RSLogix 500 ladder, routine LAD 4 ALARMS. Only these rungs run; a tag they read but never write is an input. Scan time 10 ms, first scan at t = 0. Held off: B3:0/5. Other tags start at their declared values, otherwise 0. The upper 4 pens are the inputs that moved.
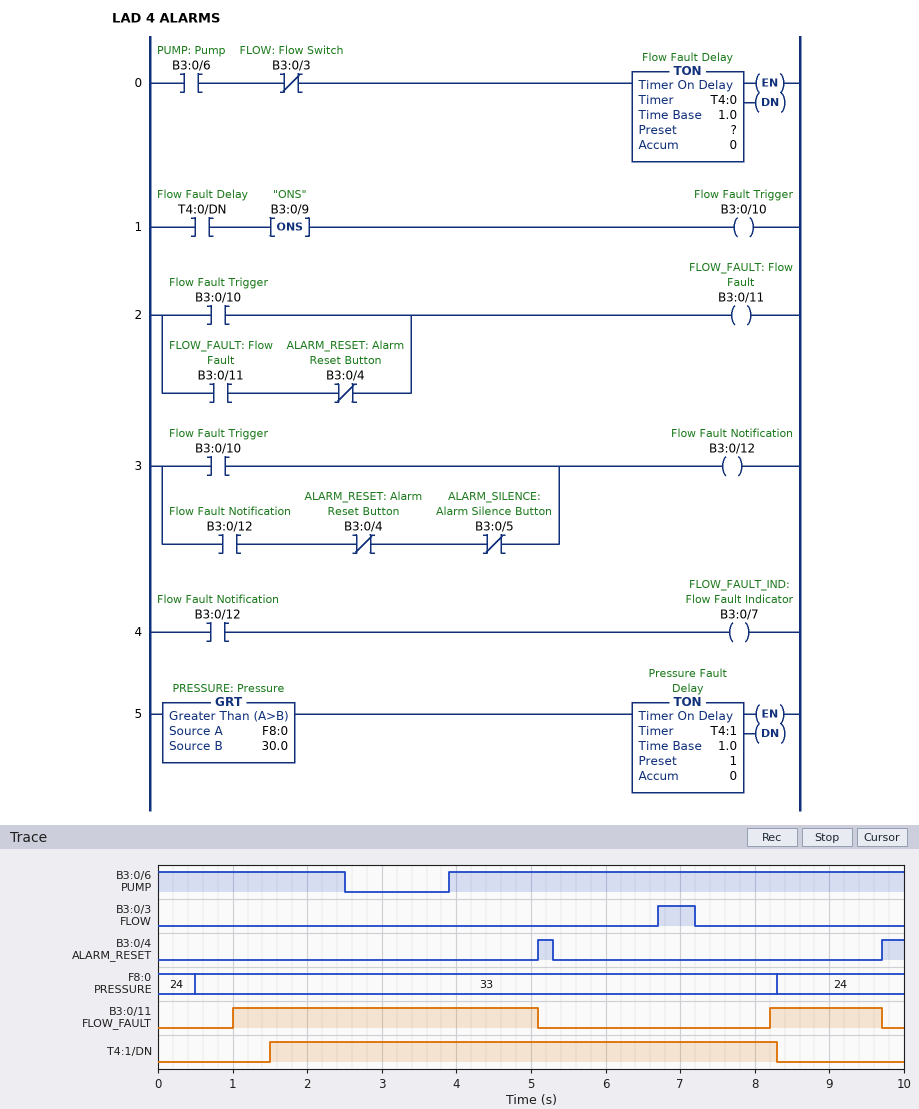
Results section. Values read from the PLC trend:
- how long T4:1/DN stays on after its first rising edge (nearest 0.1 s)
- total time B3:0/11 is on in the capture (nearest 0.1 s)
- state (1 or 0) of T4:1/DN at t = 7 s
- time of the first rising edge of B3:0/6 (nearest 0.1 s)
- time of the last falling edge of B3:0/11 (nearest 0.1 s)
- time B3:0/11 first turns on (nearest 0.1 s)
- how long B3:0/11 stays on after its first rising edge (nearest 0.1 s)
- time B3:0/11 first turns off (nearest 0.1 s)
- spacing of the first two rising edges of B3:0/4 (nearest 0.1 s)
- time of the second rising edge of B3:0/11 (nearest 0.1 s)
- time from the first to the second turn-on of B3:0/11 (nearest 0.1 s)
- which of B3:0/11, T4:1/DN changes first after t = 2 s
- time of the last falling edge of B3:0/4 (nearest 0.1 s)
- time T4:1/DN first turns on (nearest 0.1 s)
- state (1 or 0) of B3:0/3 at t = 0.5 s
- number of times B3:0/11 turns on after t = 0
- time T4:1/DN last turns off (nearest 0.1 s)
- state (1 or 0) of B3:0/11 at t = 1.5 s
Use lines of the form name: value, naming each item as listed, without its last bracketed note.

how long T4:1/DN stays on after its first rising edge: 6.8 s
total time B3:0/11 is on in the capture: 5.6 s
state (1 or 0) of T4:1/DN at t = 7 s: 1
time of the first rising edge of B3:0/6: 3.9 s
time of the last falling edge of B3:0/11: 9.7 s
time B3:0/11 first turns on: 1.0 s
how long B3:0/11 stays on after its first rising edge: 4.1 s
time B3:0/11 first turns off: 5.1 s
spacing of the first two rising edges of B3:0/4: 4.6 s
time of the second rising edge of B3:0/11: 8.2 s
time from the first to the second turn-on of B3:0/11: 7.2 s
which of B3:0/11, T4:1/DN changes first after t = 2 s: B3:0/11
time of the last falling edge of B3:0/4: 5.3 s
time T4:1/DN first turns on: 1.5 s
state (1 or 0) of B3:0/3 at t = 0.5 s: 0
number of times B3:0/11 turns on after t = 0: 2
time T4:1/DN last turns off: 8.3 s
state (1 or 0) of B3:0/11 at t = 1.5 s: 1
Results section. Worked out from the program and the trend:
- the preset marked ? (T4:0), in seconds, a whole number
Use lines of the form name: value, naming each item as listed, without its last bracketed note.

the preset marked ? (T4:0), in seconds, a whole number: 1 s
